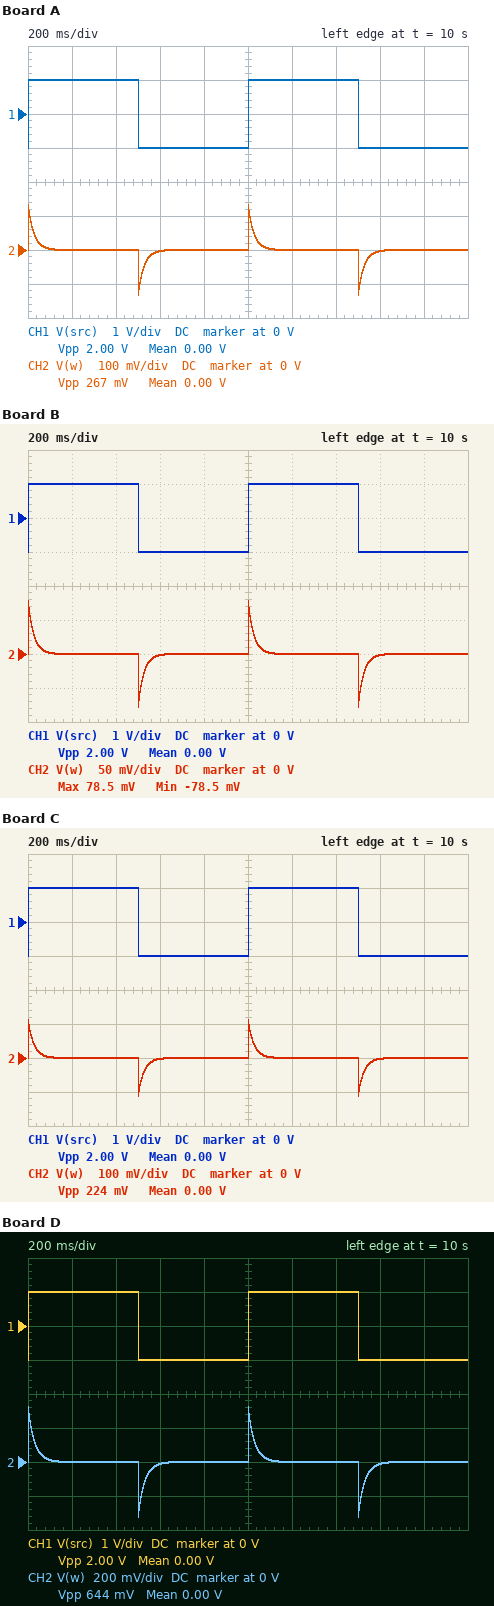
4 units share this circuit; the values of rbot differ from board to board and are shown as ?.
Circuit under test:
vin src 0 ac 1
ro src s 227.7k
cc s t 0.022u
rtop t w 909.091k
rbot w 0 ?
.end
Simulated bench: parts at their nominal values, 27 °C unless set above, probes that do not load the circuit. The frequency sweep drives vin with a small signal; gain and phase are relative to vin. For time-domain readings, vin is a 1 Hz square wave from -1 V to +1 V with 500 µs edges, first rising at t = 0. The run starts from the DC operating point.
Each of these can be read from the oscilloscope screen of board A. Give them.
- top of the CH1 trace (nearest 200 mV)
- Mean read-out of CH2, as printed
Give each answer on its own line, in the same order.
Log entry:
1.0 V
0.00 V
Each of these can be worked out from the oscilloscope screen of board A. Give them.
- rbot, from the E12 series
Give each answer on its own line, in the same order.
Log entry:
82 kΩ
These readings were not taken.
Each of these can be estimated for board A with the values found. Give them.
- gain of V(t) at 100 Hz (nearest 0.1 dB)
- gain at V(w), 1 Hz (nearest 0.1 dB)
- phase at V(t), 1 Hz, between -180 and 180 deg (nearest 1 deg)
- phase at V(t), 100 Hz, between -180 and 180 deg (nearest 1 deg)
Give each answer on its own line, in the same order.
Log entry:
-1.8 dB
-39.0 dB
80 deg
3 deg
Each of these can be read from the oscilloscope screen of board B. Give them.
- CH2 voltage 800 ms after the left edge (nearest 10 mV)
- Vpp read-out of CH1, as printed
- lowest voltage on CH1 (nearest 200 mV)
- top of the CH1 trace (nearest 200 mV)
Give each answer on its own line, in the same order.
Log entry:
0 V
2.00 V
-1.0 V
1.0 V
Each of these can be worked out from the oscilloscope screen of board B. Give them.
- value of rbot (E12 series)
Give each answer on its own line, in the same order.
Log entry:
47 kΩ
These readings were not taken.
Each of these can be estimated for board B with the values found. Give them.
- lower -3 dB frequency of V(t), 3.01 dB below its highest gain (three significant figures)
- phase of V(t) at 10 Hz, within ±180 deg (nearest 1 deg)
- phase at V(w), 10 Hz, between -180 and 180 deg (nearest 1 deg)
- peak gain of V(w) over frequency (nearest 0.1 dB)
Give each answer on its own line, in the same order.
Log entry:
6.11 Hz
31 deg
31 deg
-28.0 dB
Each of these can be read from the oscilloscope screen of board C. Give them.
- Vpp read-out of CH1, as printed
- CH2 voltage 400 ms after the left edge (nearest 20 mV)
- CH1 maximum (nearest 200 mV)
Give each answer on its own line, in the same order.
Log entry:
2.00 V
0 V
1.0 V
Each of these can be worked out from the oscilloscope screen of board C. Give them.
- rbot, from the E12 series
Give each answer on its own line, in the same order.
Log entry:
68 kΩ
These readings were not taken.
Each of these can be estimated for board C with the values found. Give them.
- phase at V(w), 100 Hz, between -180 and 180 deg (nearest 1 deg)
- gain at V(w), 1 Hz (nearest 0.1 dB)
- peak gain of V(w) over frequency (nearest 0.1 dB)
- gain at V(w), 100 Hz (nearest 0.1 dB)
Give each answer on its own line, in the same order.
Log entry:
3 deg
-40.7 dB
-25.0 dB
-25.0 dB
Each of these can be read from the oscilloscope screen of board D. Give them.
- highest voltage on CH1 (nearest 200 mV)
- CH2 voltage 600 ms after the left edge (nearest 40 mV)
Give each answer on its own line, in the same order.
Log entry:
1.0 V
0 V
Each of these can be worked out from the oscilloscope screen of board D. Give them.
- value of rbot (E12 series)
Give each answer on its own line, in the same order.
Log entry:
220 kΩ
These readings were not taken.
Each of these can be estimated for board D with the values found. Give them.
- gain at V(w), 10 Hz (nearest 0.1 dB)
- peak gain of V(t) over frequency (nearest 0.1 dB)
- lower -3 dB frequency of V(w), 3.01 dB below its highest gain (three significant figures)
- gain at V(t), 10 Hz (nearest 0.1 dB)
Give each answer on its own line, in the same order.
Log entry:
-16.9 dB
-1.6 dB
5.33 Hz
-2.7 dB
